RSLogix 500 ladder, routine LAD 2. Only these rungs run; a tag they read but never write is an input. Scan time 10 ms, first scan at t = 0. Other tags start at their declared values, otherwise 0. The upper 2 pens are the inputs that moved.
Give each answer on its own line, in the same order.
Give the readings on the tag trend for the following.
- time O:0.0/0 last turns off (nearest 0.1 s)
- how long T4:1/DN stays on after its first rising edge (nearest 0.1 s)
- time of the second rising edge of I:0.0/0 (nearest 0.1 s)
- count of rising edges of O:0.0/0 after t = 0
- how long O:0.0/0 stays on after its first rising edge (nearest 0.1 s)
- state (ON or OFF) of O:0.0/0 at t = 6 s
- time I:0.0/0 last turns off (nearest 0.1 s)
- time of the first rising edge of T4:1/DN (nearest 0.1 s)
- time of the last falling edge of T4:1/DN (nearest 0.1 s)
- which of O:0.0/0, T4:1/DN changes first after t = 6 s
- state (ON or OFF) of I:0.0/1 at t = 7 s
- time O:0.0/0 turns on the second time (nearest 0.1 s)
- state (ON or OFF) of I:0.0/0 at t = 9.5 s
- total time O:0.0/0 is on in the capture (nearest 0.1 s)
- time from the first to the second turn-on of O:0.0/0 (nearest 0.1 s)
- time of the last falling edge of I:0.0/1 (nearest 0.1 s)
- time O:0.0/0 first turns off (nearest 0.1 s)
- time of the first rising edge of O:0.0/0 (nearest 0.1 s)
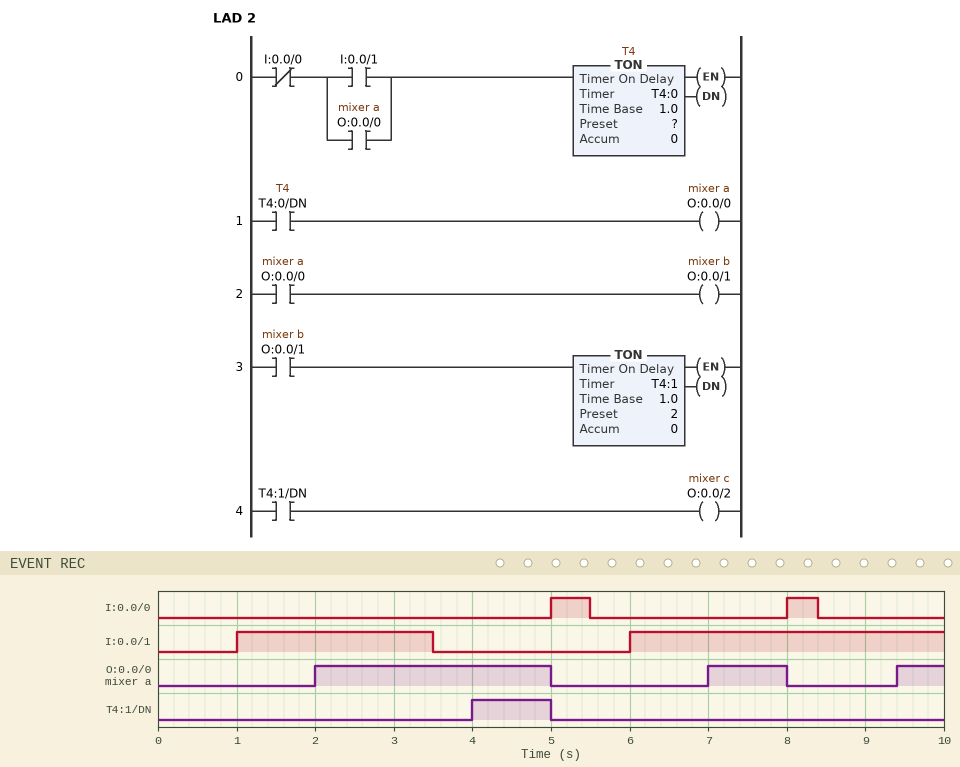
8.0 s
1.0 s
8.0 s
3
3.0 s
OFF
8.4 s
4.0 s
5.0 s
O:0.0/0
ON
7.0 s
OFF
4.6 s
5.0 s
3.5 s
5.0 s
2.0 s
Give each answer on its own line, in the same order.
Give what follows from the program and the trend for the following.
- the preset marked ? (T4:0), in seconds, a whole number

1 s
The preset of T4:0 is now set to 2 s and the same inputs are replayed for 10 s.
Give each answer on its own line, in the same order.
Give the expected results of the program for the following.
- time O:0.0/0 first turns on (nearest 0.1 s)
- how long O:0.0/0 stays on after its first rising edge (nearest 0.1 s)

3.0 s
2.0 s
